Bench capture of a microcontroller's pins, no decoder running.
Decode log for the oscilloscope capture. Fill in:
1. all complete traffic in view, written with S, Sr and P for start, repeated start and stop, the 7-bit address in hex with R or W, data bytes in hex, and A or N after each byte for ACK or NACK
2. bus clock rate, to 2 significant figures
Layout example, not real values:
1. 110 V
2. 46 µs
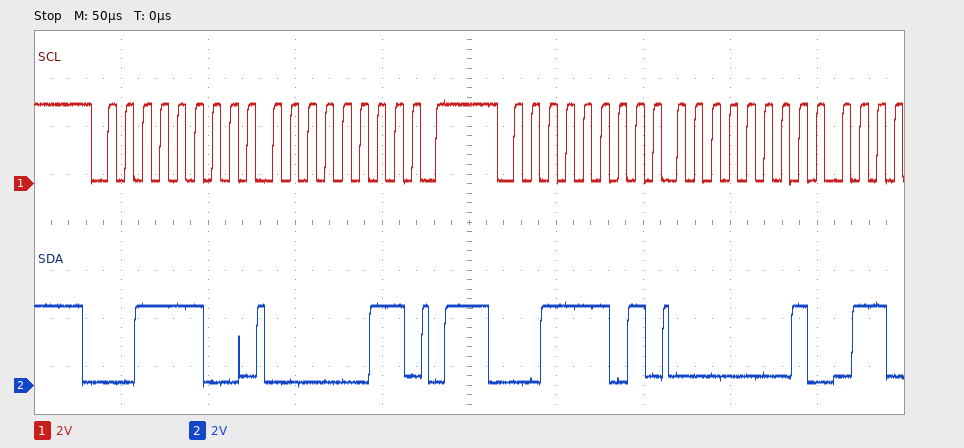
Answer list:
1. S 1EW A 03 A P S 1ER A 01 A
2. 100 kHz
